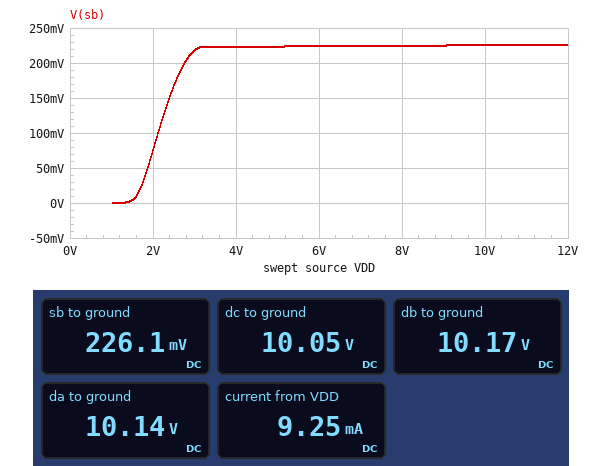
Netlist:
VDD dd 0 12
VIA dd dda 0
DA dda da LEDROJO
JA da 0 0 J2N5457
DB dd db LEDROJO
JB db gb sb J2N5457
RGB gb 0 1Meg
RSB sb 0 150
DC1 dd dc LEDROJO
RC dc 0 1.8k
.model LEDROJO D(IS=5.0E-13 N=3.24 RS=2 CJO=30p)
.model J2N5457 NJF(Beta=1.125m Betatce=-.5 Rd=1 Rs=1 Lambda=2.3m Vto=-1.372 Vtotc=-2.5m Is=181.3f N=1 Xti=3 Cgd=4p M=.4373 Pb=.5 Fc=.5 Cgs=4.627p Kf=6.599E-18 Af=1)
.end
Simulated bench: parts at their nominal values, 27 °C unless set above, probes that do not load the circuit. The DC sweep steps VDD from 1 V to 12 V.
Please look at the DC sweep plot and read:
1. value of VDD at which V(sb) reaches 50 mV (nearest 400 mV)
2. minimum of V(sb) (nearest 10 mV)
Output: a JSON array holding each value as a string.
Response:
["2.0 V", "0 V"]
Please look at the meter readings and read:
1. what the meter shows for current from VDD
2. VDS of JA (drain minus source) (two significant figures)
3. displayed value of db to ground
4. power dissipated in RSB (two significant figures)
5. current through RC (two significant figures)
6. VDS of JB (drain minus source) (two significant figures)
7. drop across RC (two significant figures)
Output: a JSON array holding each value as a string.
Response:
["9.25 mA", "10 V", "10.17 V", "340 µW", "5.6 mA", "9.9 V", "10 V"]
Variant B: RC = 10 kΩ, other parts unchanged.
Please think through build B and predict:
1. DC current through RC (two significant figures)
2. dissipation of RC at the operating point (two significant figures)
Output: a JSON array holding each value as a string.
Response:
["1.0 mA", "10 mW"]
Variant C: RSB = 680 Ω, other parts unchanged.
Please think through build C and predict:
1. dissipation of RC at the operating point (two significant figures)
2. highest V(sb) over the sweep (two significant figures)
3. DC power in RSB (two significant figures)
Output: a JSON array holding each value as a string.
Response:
["56 mW", "540 mV", "430 µW"]
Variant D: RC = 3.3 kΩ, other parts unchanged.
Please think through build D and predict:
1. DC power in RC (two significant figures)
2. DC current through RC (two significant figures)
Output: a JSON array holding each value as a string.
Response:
["31 mW", "3.1 mA"]
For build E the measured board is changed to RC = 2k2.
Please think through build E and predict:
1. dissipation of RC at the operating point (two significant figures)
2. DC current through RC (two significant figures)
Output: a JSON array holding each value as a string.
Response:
["46 mW", "4.6 mA"]
